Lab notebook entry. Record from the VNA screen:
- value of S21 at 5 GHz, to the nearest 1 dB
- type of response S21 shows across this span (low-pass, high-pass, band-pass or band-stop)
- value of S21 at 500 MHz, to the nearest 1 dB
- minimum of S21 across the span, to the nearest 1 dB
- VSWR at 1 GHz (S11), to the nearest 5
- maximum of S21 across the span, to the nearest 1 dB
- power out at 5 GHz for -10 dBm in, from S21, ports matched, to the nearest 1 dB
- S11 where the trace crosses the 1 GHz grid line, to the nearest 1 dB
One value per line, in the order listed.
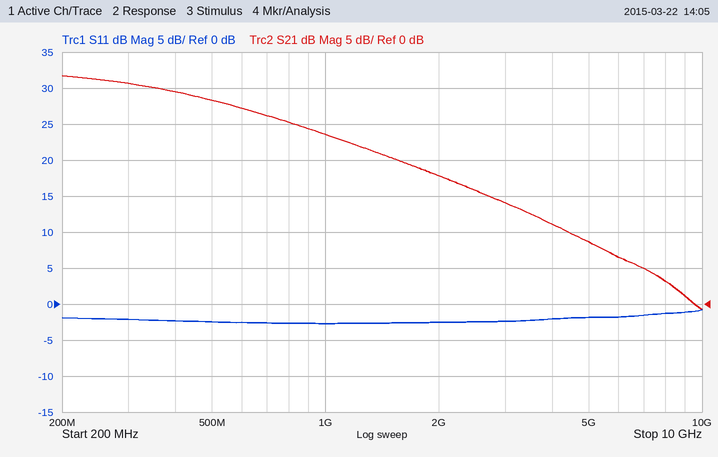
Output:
9 dB
low-pass
28 dB
-1 dB
5
32 dB
-1 dBm
-3 dB
